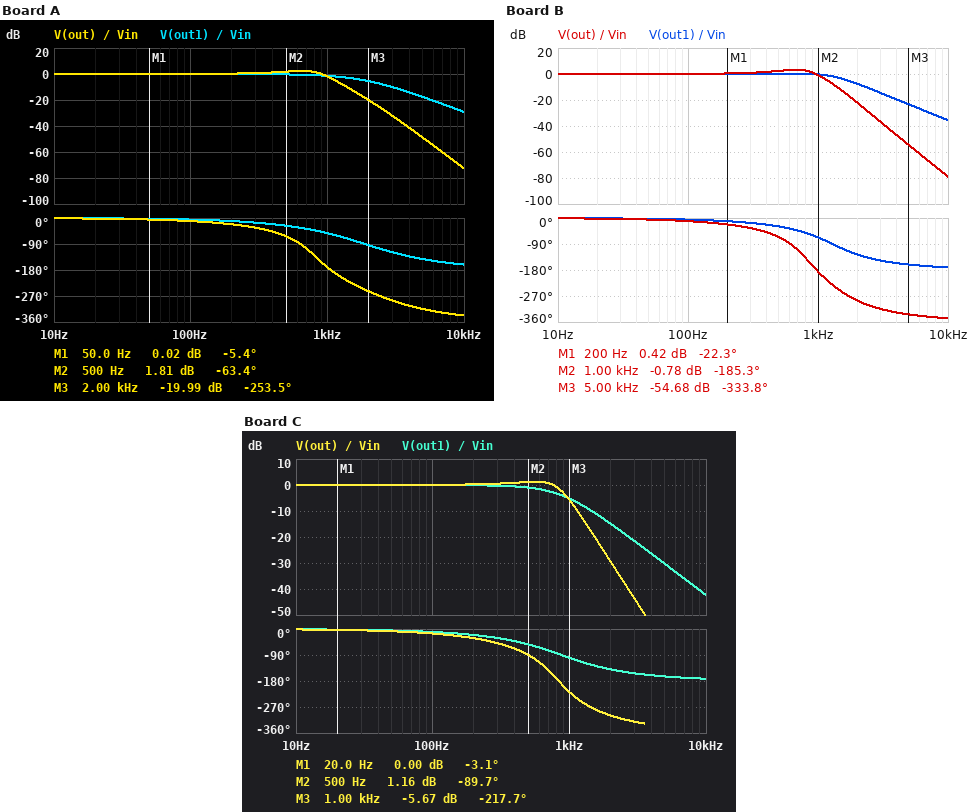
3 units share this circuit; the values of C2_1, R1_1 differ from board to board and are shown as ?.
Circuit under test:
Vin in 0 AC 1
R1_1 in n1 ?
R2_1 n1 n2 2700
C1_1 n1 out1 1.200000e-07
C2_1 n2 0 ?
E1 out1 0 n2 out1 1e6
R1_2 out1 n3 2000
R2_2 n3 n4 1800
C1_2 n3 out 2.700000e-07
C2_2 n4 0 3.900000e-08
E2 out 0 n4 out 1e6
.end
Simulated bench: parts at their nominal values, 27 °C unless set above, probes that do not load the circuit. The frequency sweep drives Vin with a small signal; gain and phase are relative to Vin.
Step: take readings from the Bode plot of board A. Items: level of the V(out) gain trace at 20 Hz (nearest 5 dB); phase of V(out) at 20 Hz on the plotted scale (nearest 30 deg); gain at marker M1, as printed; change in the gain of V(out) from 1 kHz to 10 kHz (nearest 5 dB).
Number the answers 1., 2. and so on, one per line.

1. 0 dB
2. 0 deg
3. 0.02 dB
4. -70 dB
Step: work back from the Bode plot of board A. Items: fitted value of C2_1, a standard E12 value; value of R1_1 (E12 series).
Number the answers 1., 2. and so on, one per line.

1. 47 nF
2. 470 Ω
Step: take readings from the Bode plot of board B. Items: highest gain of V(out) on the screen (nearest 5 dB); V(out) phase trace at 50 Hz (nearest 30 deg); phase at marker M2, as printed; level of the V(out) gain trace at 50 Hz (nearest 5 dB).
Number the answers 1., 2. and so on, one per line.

1. 5 dB
2. 0 deg
3. -185.3 deg
4. 0 dB
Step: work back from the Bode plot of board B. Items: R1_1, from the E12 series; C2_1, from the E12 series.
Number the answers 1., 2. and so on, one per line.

1. 1.2 kΩ
2. 39 nF
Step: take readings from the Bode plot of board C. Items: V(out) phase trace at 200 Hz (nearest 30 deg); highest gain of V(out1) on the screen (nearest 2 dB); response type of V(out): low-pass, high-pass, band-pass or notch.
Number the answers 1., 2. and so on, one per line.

1. -30 deg
2. 0 dB
3. low-pass
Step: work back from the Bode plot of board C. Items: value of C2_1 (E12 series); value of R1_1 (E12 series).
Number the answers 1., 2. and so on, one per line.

1. 68 nF
2. 1.5 kΩ
